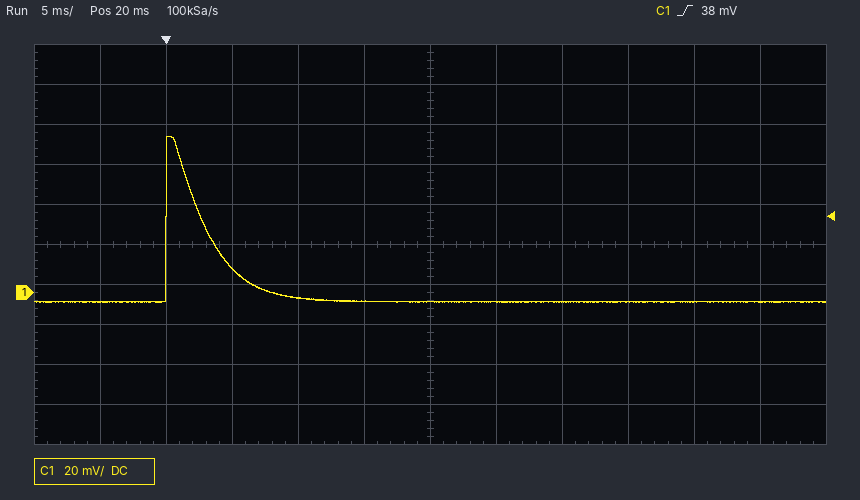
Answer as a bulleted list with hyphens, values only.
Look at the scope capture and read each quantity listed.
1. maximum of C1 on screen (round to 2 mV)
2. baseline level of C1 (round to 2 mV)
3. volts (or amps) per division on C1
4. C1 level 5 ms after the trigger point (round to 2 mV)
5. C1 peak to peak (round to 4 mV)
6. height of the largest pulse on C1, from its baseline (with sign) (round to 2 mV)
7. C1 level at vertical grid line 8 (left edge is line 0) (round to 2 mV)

- 78 mV
- -4 mV
- 20 mV
- 12 mV
- 84 mV
- +82 mV
- -4 mV
